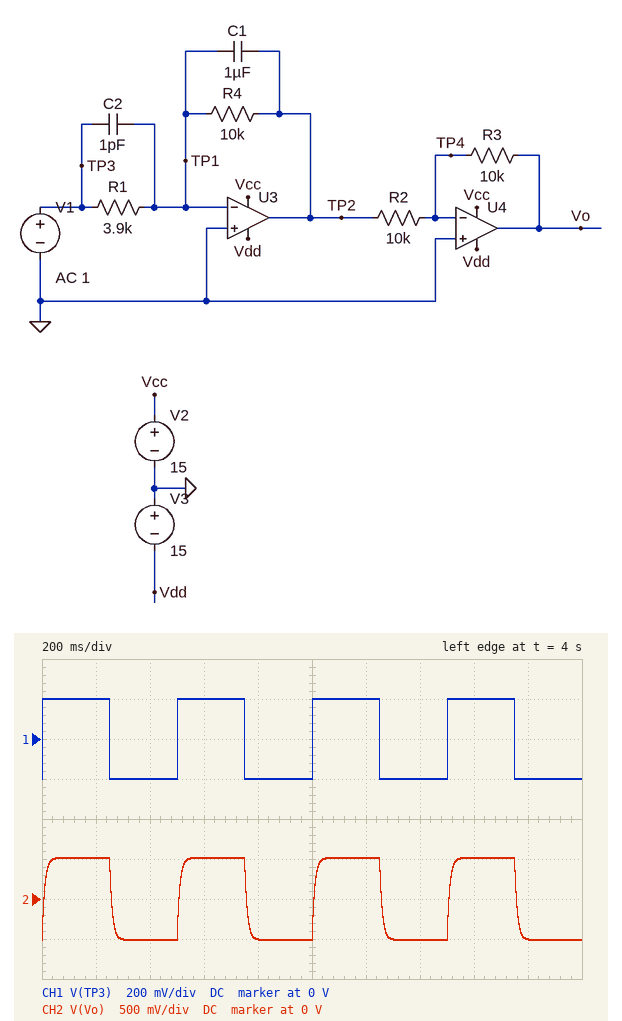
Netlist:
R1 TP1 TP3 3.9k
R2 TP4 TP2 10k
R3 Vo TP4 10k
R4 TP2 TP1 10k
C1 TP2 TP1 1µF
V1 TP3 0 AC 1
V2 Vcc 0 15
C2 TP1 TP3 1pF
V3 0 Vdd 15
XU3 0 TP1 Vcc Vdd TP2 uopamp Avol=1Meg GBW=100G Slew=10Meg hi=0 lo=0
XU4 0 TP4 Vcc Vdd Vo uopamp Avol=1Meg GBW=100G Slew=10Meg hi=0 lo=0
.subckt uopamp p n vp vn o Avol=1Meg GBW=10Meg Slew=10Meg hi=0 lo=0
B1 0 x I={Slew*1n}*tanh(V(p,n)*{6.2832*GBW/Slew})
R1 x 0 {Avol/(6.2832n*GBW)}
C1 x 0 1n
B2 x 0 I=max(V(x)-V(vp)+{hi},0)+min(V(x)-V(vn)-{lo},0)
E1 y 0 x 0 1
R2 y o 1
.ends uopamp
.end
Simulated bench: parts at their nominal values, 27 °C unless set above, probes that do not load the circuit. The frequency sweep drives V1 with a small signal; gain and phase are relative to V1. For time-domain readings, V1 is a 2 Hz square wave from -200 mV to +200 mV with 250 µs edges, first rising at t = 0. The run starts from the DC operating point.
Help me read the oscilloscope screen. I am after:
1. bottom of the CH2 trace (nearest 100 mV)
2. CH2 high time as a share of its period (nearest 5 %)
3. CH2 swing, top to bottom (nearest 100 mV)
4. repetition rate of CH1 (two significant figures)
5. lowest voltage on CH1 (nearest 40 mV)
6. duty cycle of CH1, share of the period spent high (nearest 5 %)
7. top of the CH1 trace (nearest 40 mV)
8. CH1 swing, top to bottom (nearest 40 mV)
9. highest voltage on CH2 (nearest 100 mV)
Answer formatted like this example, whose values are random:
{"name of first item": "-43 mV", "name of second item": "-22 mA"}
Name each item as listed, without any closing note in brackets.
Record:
{"bottom of the CH2 trace": "-500 mV", "CH2 high time as a share of its period": "50 %", "CH2 swing, top to bottom": "1.0 V", "repetition rate of CH1": "2.0 Hz", "lowest voltage on CH1": "-200 mV", "duty cycle of CH1, share of the period spent high": "50 %", "top of the CH1 trace": "200 mV", "CH1 swing, top to bottom": "400 mV", "highest voltage on CH2": "500 mV"}
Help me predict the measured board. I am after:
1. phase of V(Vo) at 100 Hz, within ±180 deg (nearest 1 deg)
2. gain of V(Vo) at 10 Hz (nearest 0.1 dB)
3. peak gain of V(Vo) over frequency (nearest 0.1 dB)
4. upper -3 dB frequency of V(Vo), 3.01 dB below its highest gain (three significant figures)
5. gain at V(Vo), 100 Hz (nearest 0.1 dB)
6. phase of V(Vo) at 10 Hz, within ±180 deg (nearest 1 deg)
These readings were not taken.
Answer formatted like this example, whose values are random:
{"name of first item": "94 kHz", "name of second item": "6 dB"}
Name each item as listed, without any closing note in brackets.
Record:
{"phase of V(Vo) at 100 Hz, within ±180 deg": "-81 deg", "gain of V(Vo) at 10 Hz": "6.7 dB", "peak gain of V(Vo) over frequency": "8.2 dB", "upper -3 dB frequency of V(Vo), 3.01 dB below its highest gain": "15.9 Hz", "gain at V(Vo), 100 Hz": "-7.9 dB", "phase of V(Vo) at 10 Hz, within ±180 deg": "-32 deg"}
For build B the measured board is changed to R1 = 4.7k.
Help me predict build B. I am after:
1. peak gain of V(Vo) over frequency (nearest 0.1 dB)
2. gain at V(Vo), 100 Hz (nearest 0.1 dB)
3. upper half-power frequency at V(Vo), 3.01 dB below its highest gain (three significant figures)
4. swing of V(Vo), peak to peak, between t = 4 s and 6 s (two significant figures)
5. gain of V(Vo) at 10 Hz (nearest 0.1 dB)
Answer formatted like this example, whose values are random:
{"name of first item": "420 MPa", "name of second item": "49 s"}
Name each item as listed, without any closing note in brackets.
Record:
{"peak gain of V(Vo) over frequency": "6.6 dB", "gain at V(Vo), 100 Hz": "-9.5 dB", "upper half-power frequency at V(Vo), 3.01 dB below its highest gain": "15.9 Hz", "swing of V(Vo), peak to peak, between t = 4 s and 6 s": "850 mV", "gain of V(Vo) at 10 Hz": "5.1 dB"}
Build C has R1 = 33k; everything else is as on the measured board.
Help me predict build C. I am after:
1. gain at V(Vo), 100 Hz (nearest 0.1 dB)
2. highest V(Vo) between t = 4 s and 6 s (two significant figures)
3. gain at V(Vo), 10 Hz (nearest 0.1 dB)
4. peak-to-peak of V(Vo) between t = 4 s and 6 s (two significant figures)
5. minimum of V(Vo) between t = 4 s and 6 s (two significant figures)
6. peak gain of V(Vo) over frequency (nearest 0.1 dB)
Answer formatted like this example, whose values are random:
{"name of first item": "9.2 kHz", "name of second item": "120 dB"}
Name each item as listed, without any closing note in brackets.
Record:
{"gain at V(Vo), 100 Hz": "-26.4 dB", "highest V(Vo) between t = 4 s and 6 s": "61 mV", "gain at V(Vo), 10 Hz": "-11.8 dB", "peak-to-peak of V(Vo) between t = 4 s and 6 s": "120 mV", "minimum of V(Vo) between t = 4 s and 6 s": "-61 mV", "peak gain of V(Vo) over frequency": "-10.4 dB"}
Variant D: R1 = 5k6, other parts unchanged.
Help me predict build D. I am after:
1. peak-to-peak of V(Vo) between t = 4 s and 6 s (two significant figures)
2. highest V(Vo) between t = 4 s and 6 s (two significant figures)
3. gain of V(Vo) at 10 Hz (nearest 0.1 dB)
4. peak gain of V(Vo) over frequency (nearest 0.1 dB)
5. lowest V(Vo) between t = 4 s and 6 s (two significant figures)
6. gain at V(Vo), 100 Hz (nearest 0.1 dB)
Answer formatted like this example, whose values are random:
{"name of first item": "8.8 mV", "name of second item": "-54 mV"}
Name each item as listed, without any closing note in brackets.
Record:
{"peak-to-peak of V(Vo) between t = 4 s and 6 s": "710 mV", "highest V(Vo) between t = 4 s and 6 s": "360 mV", "gain of V(Vo) at 10 Hz": "3.6 dB", "peak gain of V(Vo) over frequency": "5.0 dB", "lowest V(Vo) between t = 4 s and 6 s": "-360 mV", "gain at V(Vo), 100 Hz": "-11.0 dB"}
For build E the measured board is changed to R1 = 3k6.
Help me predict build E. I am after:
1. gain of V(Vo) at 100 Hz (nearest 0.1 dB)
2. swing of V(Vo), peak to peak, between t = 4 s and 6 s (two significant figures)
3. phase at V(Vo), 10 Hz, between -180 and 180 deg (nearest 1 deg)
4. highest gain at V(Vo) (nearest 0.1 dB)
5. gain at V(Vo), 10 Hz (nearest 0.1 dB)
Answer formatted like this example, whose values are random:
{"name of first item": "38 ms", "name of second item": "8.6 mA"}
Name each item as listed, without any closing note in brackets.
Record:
{"gain of V(Vo) at 100 Hz": "-7.2 dB", "swing of V(Vo), peak to peak, between t = 4 s and 6 s": "1.1 V", "phase at V(Vo), 10 Hz, between -180 and 180 deg": "-32 deg", "highest gain at V(Vo)": "8.9 dB", "gain at V(Vo), 10 Hz": "7.4 dB"}
